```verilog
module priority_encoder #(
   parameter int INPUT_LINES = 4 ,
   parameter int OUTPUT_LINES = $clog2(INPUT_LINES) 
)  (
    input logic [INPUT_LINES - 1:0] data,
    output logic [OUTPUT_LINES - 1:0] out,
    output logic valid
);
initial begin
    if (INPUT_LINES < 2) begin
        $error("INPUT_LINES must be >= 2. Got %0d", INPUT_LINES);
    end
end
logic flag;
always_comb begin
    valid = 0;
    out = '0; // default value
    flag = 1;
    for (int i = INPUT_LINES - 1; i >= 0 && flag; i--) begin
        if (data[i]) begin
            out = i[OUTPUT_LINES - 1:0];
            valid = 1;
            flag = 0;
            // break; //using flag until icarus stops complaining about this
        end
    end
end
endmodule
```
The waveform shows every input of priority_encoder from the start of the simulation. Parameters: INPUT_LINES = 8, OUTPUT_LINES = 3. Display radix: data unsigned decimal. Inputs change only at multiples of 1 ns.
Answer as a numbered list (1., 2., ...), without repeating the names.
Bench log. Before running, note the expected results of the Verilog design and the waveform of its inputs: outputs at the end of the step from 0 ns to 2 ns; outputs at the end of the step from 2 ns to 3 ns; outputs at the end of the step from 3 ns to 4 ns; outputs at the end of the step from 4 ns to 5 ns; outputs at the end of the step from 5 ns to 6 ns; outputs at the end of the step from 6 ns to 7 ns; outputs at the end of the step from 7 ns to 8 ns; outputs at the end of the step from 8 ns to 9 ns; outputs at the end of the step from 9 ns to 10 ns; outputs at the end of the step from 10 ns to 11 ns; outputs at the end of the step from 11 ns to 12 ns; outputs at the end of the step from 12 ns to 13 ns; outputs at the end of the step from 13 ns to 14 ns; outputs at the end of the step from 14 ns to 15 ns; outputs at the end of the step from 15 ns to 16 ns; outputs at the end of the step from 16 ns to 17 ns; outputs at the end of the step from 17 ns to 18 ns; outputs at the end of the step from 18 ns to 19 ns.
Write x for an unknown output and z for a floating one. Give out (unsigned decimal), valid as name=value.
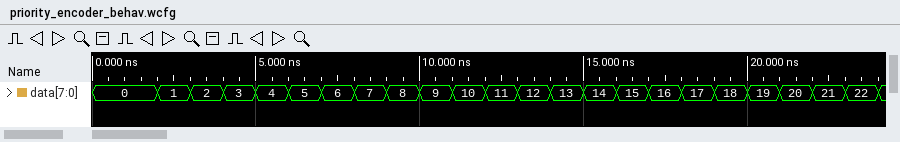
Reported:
1. out=0, valid=0
2. out=0, valid=1
3. out=1, valid=1
4. out=1, valid=1
5. out=2, valid=1
6. out=2, valid=1
7. out=2, valid=1
8. out=2, valid=1
9. out=3, valid=1
10. out=3, valid=1
11. out=3, valid=1
12. out=3, valid=1
13. out=3, valid=1
14. out=3, valid=1
15. out=3, valid=1
16. out=3, valid=1
17. out=4, valid=1
18. out=4, valid=1
